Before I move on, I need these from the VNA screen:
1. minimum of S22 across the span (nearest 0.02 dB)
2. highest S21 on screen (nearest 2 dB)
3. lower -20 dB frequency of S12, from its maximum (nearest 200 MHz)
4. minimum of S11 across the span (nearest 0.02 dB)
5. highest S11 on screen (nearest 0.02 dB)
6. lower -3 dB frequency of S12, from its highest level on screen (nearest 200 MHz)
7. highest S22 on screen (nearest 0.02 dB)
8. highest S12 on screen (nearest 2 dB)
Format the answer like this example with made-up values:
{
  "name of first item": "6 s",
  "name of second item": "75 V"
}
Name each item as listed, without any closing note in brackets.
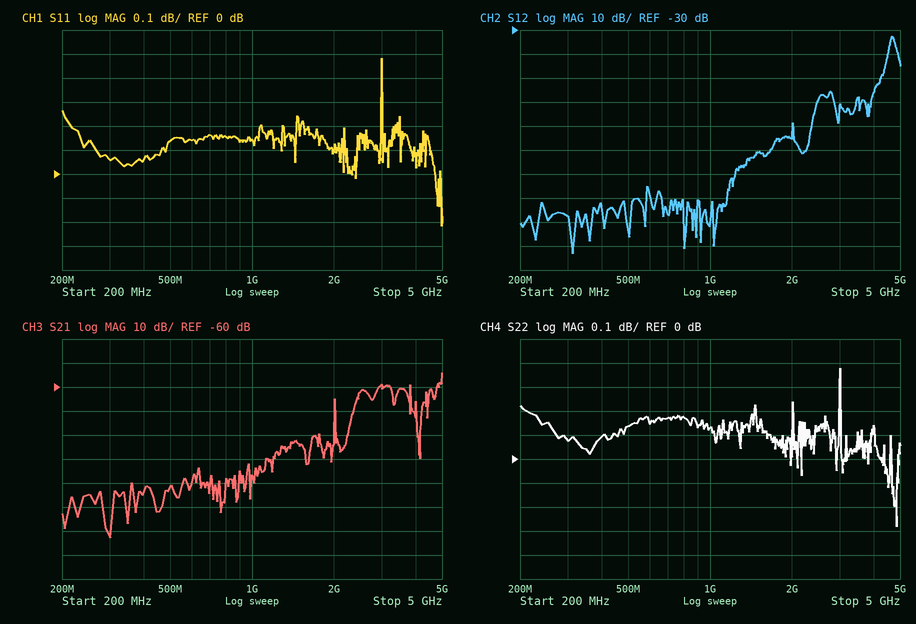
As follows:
{
  "minimum of S22 across the span": "-0.28 dB",
  "highest S21 on screen": "-54 dB",
  "lower -20 dB frequency of S12, from its maximum": "4.2 GHz",
  "minimum of S11 across the span": "-0.22 dB",
  "highest S11 on screen": "0.48 dB",
  "lower -3 dB frequency of S12, from its highest level on screen": "4.6 GHz",
  "highest S22 on screen": "0.38 dB",
  "highest S12 on screen": "-32 dB"
}
